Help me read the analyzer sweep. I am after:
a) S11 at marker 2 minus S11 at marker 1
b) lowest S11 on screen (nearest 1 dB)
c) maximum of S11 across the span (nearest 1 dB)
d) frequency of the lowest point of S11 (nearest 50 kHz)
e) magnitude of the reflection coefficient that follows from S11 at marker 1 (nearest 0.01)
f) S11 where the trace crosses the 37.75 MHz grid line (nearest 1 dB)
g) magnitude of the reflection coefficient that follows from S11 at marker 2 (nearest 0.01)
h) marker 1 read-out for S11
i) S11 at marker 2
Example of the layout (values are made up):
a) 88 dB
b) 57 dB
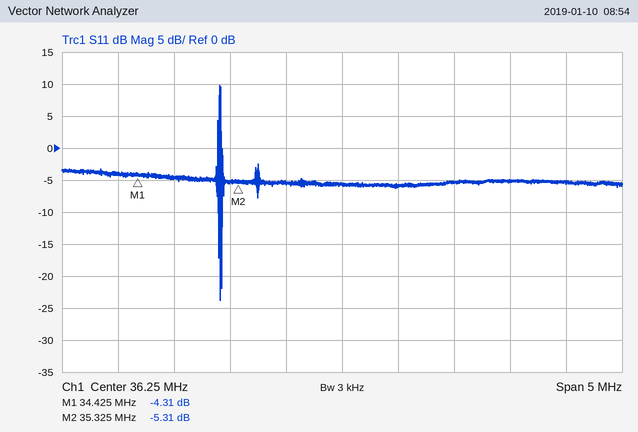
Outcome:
a) -1.00 dB
b) -24 dB
c) 10 dB
d) 35.15 MHz
e) 0.61
f) -5 dB
g) 0.54
h) -4.31 dB
i) -5.31 dB
